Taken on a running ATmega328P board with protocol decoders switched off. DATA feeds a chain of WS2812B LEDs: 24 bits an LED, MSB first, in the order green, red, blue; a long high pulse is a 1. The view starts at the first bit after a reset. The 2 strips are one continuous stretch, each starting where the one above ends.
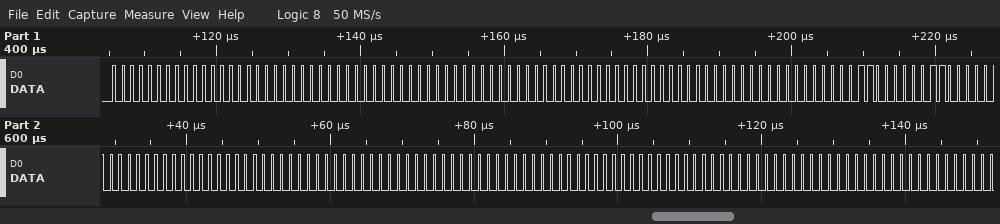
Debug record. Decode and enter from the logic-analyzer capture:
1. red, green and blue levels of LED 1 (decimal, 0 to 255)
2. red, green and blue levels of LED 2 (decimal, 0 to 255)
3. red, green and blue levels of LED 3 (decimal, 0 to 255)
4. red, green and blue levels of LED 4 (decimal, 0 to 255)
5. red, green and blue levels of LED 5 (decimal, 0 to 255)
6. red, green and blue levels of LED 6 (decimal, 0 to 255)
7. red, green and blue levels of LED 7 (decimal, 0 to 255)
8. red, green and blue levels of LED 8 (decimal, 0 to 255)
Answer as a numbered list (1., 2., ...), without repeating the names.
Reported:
1. 0, 0, 0
2. 0, 0, 0
3. 0, 0, 0
4. 24, 0, 24
5. 0, 0, 0
6. 0, 0, 0
7. 0, 0, 0
8. 0, 0, 0
